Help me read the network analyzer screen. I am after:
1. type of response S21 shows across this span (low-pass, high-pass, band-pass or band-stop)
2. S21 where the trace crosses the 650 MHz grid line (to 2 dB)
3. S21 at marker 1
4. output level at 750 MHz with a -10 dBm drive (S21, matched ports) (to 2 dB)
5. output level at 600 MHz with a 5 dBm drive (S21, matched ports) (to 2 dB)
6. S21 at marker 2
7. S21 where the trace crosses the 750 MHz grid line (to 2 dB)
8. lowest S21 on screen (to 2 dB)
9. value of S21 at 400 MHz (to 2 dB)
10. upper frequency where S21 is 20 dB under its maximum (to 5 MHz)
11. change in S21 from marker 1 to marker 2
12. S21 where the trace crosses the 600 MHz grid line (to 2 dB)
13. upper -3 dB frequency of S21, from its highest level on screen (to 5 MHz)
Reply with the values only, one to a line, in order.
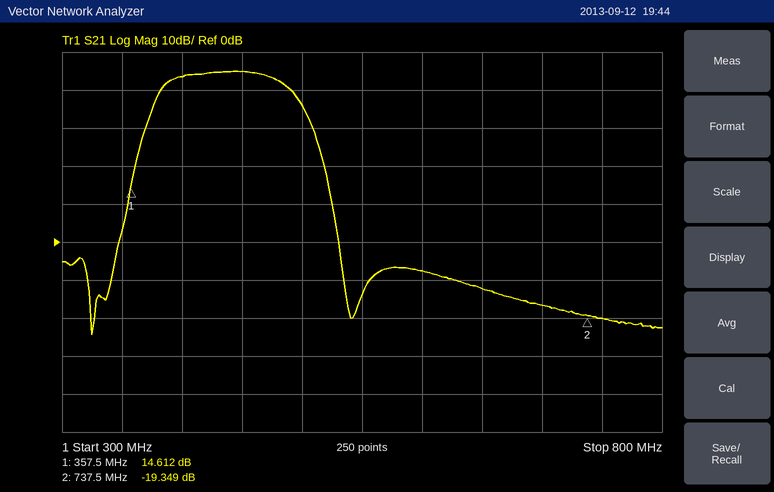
band-pass
-12 dB
14.612 dB
-30 dBm
-2 dBm
-19.349 dB
-20 dB
-24 dB
44 dB
515 MHz
-33.961 dB
-8 dB
485 MHz
